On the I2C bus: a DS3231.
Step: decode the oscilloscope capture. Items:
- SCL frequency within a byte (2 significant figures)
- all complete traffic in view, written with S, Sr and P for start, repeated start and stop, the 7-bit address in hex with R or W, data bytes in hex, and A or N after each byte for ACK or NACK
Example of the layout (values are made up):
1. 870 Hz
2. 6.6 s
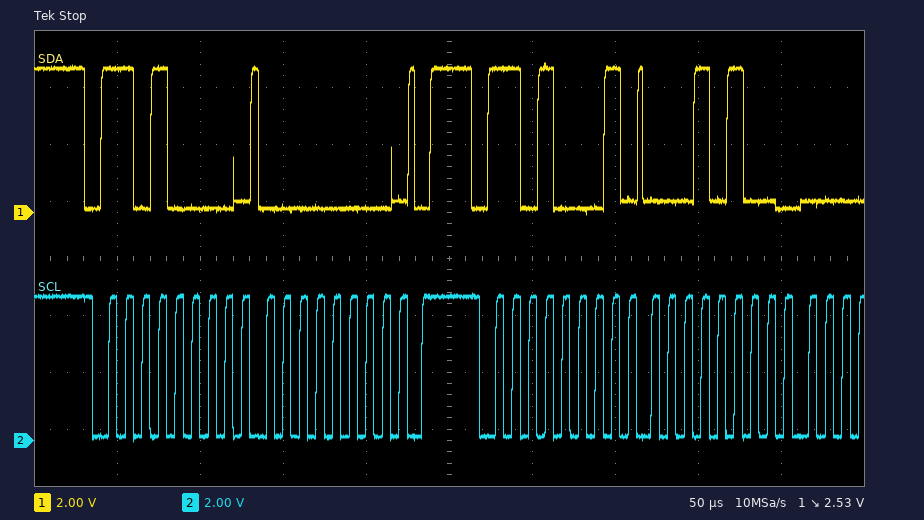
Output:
1. 100 kHz
2. S 68W A 00 A P S 68R A 14 A
